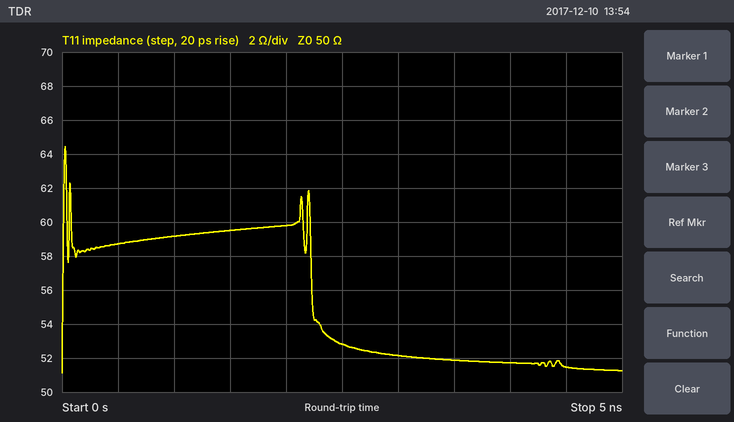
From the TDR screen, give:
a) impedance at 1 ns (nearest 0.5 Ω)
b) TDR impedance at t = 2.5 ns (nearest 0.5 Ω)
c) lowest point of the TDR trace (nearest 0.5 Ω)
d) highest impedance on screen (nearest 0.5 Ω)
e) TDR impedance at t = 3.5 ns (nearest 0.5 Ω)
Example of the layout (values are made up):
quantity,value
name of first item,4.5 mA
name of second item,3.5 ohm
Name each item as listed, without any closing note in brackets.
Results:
quantity,value
impedance at 1 ns,59.0 Ω
TDR impedance at t = 2.5 ns,53.0 Ω
lowest point of the TDR trace,51.0 Ω
highest impedance on screen,64.5 Ω
TDR impedance at t = 3.5 ns,52.0 Ω
